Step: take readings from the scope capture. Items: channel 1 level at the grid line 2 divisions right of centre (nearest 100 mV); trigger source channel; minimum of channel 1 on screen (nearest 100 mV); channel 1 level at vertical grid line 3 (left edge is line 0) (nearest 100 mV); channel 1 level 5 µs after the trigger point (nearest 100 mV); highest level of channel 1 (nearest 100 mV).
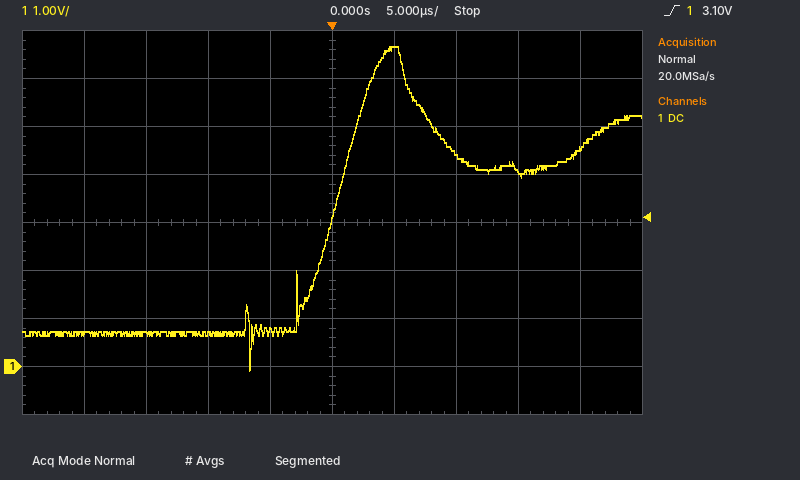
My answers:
4.4 V
channel 1
-100 mV
700 mV
6.6 V
6.7 V
